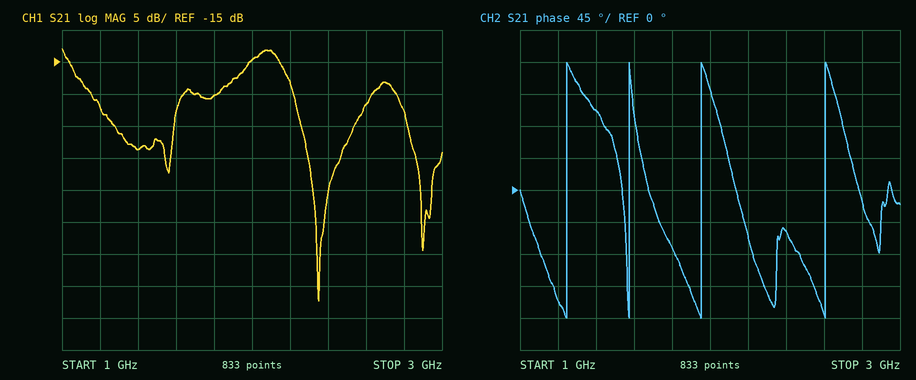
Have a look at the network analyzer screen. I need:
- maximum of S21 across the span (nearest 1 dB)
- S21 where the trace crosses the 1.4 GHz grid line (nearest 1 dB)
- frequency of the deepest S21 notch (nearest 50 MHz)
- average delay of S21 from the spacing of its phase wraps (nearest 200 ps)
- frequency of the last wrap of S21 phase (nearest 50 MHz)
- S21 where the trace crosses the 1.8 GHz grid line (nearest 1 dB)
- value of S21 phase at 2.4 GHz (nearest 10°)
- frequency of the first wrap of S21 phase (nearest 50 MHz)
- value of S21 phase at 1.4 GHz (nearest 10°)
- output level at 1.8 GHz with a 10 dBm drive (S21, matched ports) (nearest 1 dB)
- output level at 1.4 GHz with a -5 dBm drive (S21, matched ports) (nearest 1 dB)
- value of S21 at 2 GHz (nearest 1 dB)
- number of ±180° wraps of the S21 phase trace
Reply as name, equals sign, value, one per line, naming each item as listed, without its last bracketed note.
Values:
maximum of S21 across the span = -13 dB
S21 where the trace crosses the 1.4 GHz grid line = -29 dB
frequency of the deepest S21 notch = 2.35 GHz
average delay of S21 from the spacing of its phase wraps = 2.2 ns
frequency of the last wrap of S21 phase = 2.60 GHz
S21 where the trace crosses the 1.8 GHz grid line = -20 dB
value of S21 phase at 2.4 GHz = -60°
frequency of the first wrap of S21 phase = 1.25 GHz
value of S21 phase at 1.4 GHz = 110°
output level at 1.8 GHz with a 10 dBm drive (S21, matched ports) = -10 dBm
output level at 1.4 GHz with a -5 dBm drive (S21, matched ports) = -34 dBm
value of S21 at 2 GHz = -15 dB
number of ±180° wraps of the S21 phase trace = 4
